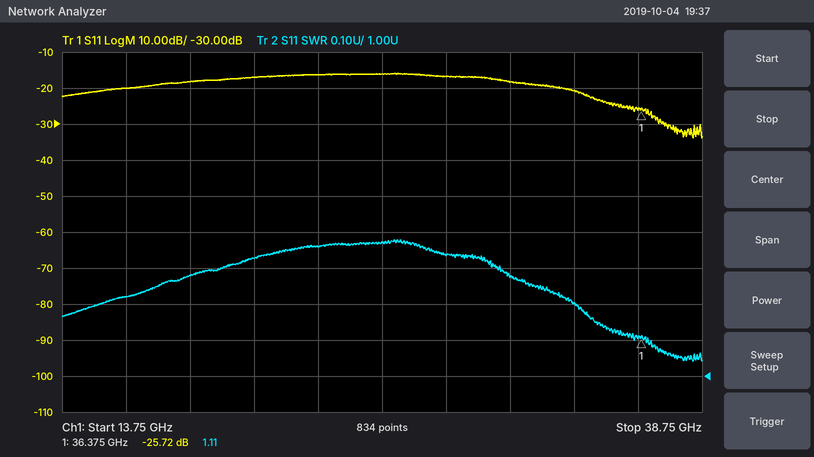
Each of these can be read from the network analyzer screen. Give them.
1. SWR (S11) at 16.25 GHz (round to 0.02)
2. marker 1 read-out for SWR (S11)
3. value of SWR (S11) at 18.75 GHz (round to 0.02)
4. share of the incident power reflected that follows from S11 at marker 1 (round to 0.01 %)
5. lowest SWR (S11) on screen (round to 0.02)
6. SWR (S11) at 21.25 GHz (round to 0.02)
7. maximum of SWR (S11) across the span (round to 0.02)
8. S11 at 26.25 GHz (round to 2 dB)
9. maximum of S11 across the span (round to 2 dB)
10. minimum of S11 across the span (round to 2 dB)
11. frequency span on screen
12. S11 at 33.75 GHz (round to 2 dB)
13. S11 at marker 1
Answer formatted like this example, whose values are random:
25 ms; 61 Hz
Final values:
1.22; 1.11; 1.28; 0.27 %; 1.04; 1.32; 1.38; -16 dB; -16 dB; -34 dB; 25 GHz; -20 dB; -25.72 dB
